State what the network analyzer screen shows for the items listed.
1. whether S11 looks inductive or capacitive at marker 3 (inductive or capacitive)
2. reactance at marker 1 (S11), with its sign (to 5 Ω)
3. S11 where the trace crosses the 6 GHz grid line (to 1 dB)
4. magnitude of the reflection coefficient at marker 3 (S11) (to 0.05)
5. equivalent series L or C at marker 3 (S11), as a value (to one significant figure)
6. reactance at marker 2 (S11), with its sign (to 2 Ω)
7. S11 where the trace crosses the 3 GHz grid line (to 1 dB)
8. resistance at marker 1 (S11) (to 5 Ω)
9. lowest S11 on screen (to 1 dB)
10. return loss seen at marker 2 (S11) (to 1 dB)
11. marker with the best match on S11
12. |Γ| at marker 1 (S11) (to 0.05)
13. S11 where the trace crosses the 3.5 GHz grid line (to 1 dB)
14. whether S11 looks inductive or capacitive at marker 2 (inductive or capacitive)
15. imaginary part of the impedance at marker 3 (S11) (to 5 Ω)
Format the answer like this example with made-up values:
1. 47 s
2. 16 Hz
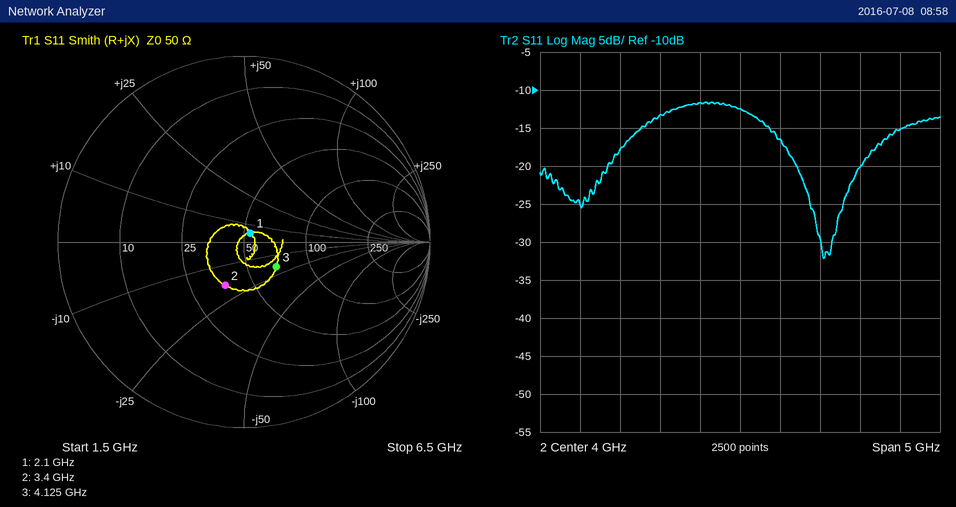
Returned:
1. capacitive
2. +5 Ω
3. -15 dB
4. 0.20
5. 2 pF
6. -18 Ω
7. -13 dB
8. 55 Ω
9. -32 dB
10. 12 dB
11. marker 1
12. 0.05
13. -12 dB
14. capacitive
15. -20 Ω
